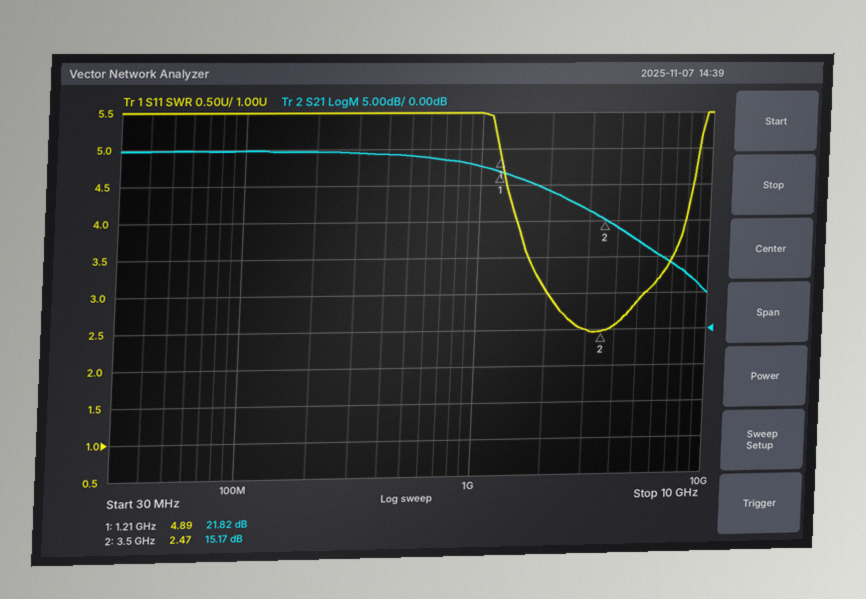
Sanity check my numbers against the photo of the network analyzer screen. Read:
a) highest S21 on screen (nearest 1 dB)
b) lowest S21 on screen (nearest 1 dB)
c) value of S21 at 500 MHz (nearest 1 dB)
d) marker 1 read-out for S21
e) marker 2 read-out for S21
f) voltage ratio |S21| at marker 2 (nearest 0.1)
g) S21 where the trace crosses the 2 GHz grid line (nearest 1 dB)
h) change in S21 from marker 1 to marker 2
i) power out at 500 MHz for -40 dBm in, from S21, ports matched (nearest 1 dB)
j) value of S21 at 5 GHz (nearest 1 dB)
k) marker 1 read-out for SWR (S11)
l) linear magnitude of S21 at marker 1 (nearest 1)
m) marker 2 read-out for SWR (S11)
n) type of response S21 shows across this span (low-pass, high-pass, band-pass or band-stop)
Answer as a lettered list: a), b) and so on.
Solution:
a) 25 dB
b) 5 dB
c) 24 dB
d) 21.82 dB
e) 15.17 dB
f) 5.7
g) 19 dB
h) -6.65 dB
i) -16 dBm
j) 12 dB
k) 4.89
l) 12
m) 2.47
n) low-pass
